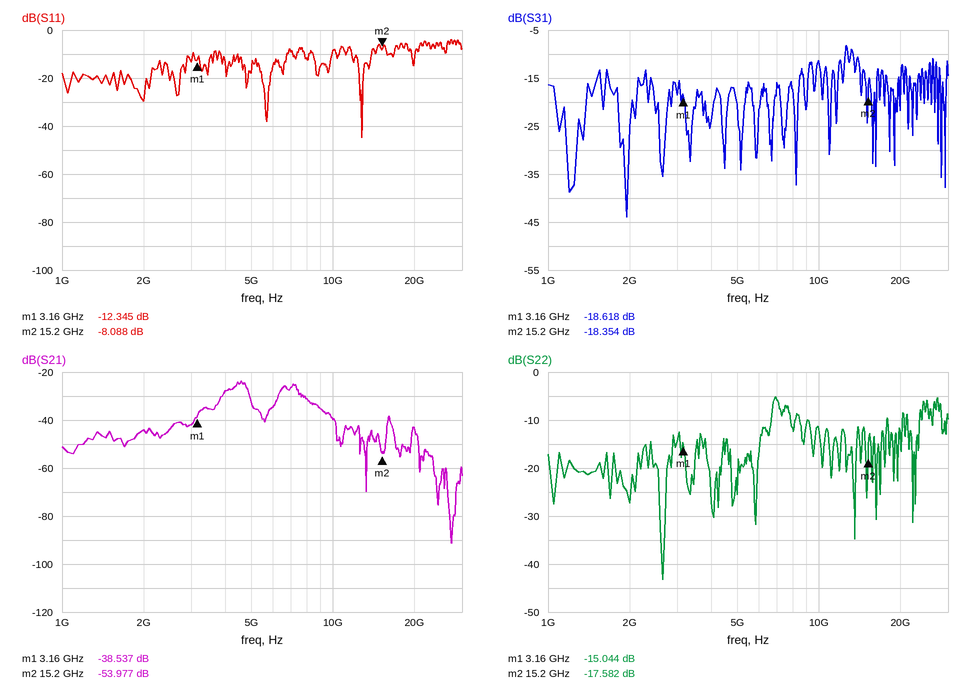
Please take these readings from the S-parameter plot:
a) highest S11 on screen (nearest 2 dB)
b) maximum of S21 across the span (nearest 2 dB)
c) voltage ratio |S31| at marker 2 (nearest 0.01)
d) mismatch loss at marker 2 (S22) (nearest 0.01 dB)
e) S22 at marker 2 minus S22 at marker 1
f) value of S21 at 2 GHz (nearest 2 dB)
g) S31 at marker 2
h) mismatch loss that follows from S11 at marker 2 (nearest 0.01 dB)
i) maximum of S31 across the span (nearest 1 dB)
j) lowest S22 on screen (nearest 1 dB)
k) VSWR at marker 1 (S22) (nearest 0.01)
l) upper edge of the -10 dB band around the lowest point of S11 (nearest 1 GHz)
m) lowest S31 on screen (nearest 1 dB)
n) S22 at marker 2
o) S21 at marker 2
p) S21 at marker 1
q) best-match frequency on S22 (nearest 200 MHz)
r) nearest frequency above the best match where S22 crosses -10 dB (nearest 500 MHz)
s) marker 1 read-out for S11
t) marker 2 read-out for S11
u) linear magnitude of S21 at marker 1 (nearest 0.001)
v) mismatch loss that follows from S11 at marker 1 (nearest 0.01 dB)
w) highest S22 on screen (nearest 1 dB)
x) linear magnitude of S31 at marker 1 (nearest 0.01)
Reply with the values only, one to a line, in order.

-4 dB
-24 dB
0.12
0.08 dB
-2.538 dB
-44 dB
-18.354 dB
0.73 dB
-8 dB
-43 dB
1.43
14 GHz
-44 dB
-17.582 dB
-53.977 dB
-38.537 dB
2.6 GHz
6.5 GHz
-12.345 dB
-8.088 dB
0.012
0.26 dB
-5 dB
0.12
